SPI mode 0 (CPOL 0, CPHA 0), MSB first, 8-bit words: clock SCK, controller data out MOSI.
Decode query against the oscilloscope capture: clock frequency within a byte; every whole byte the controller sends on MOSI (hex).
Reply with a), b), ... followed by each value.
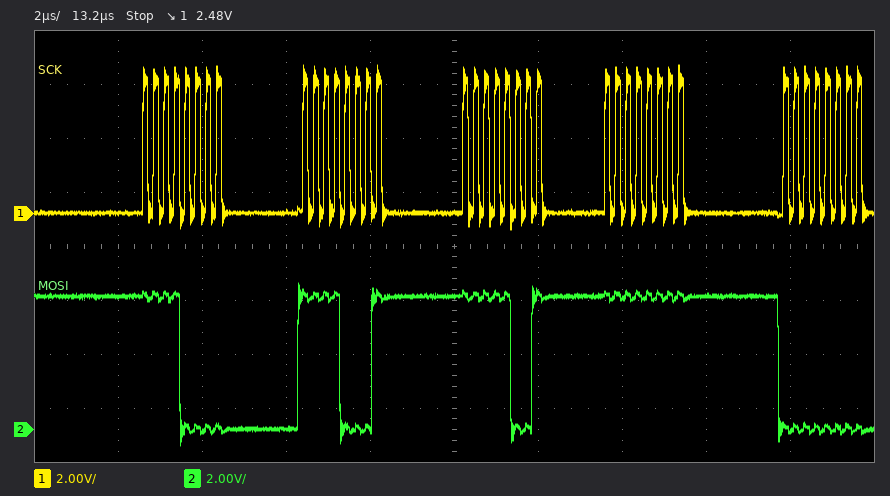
a) 4 MHz
b) F0 F1 F9 FF 00
